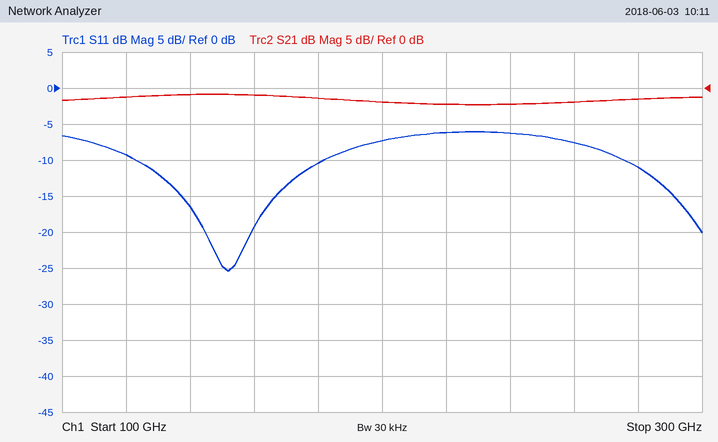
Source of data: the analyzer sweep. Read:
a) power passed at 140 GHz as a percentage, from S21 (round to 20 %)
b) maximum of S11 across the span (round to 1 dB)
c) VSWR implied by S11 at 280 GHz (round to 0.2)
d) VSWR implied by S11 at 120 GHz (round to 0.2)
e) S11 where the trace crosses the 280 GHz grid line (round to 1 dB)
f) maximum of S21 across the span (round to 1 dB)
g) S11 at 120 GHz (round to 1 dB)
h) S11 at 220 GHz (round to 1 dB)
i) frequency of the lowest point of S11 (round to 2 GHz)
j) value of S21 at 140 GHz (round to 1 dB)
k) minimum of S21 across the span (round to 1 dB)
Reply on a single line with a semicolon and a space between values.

80 %; -6 dB; 1.8; 2.0; -11 dB; -1 dB; -9 dB; -6 dB; 152 GHz; -1 dB; -2 dB
